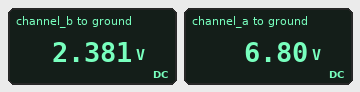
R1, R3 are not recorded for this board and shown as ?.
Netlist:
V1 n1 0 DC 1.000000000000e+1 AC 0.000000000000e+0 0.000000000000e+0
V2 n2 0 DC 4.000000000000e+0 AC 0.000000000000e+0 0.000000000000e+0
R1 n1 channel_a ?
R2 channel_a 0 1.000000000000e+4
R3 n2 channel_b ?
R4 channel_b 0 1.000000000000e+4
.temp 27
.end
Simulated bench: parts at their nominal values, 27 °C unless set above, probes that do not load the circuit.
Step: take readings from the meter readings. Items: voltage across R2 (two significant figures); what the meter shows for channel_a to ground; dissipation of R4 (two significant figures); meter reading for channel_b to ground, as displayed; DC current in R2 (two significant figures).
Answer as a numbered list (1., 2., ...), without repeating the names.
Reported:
1. 6.8 V
2. 6.80 V
3. 570 µW
4. 2.381 V
5. 680 µA
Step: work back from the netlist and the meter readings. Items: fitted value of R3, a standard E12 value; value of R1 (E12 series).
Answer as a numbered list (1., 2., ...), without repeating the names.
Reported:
1. 6.8 kΩ
2. 4.7 kΩ
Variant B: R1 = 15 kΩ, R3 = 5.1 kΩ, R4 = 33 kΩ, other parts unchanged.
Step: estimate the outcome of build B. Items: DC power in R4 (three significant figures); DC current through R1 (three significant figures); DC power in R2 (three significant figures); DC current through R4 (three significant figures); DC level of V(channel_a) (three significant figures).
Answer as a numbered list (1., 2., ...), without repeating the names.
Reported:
1. 364 µW
2. 400 µA
3. 1.60 mW
4. 105 µA
5. 4.00 V
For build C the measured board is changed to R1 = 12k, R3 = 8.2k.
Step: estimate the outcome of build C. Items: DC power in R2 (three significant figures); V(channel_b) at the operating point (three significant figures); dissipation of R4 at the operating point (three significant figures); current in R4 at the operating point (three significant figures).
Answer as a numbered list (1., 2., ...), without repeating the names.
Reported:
1. 2.07 mW
2. 2.20 V
3. 483 µW
4. 220 µA
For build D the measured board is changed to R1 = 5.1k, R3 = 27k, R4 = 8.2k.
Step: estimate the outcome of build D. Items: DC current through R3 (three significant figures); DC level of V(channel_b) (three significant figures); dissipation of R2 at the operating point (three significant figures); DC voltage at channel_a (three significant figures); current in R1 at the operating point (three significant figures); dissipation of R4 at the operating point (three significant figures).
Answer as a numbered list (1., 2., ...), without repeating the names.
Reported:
1. 114 µA
2. 932 mV
3. 4.39 mW
4. 6.62 V
5. 662 µA
6. 106 µW
